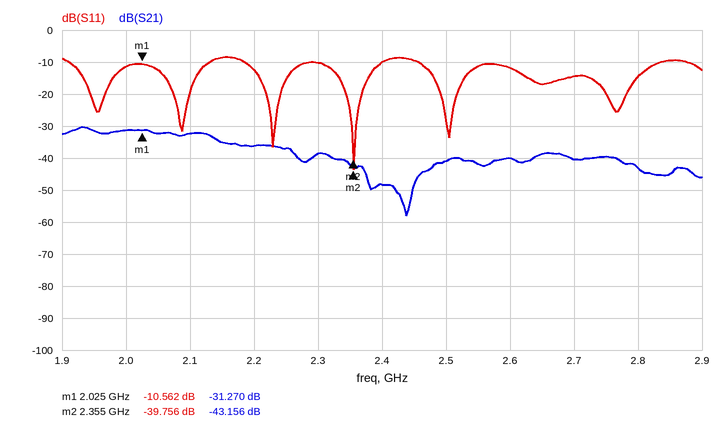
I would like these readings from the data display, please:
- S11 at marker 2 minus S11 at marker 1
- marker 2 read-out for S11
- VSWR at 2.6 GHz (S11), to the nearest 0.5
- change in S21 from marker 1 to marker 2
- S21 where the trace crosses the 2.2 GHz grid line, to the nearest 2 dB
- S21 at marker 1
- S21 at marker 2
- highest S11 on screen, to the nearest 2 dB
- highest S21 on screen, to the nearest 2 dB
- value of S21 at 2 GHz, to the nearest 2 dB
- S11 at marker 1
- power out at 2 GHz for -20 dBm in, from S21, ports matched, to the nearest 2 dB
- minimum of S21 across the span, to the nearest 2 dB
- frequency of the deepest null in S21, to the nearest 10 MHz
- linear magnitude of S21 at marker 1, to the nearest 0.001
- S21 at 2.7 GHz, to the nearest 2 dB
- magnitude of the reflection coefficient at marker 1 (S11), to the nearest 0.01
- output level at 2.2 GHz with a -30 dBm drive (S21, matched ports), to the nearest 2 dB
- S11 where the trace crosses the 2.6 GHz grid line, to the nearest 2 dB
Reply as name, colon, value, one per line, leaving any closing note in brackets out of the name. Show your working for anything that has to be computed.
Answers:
S11 at marker 2 minus S11 at marker 1: -39.756 − (-10.562) = -29.194 dB
marker 2 read-out for S11: -39.756 dB
VSWR at 2.6 GHz (S11), to the nearest 0.5: |Γ| = 10^(-12/20) = 0.2512; VSWR = (1 + 0.2512)/(1 − 0.2512) ≈ 1.67, so 1.5 to the nearest 0.5
change in S21 from marker 1 to marker 2: -43.156 − (-31.27) = -11.886 dB
S21 where the trace crosses the 2.2 GHz grid line, to the nearest 2 dB: -36 dB
S21 at marker 1: -31.270 dB
S21 at marker 2: -43.156 dB
highest S11 on screen, to the nearest 2 dB: -8 dB
highest S21 on screen, to the nearest 2 dB: -30 dB
value of S21 at 2 GHz, to the nearest 2 dB: -32 dB
S11 at marker 1: -10.562 dB
power out at 2 GHz for -20 dBm in, from S21, ports matched, to the nearest 2 dB: -20 dBm + (-32 dB) = -52 dBm
minimum of S21 across the span, to the nearest 2 dB: -58 dB
frequency of the deepest null in S21, to the nearest 10 MHz: 2.44 GHz
linear magnitude of S21 at marker 1, to the nearest 0.001: 10^(-31.27/20) ≈ 0.027
S21 at 2.7 GHz, to the nearest 2 dB: -40 dB
magnitude of the reflection coefficient at marker 1 (S11), to the nearest 0.01: 10^(-10.562/20) ≈ 0.30
output level at 2.2 GHz with a -30 dBm drive (S21, matched ports), to the nearest 2 dB: -30 dBm + (-36 dB) = -66 dBm
S11 where the trace crosses the 2.6 GHz grid line, to the nearest 2 dB: -12 dB
